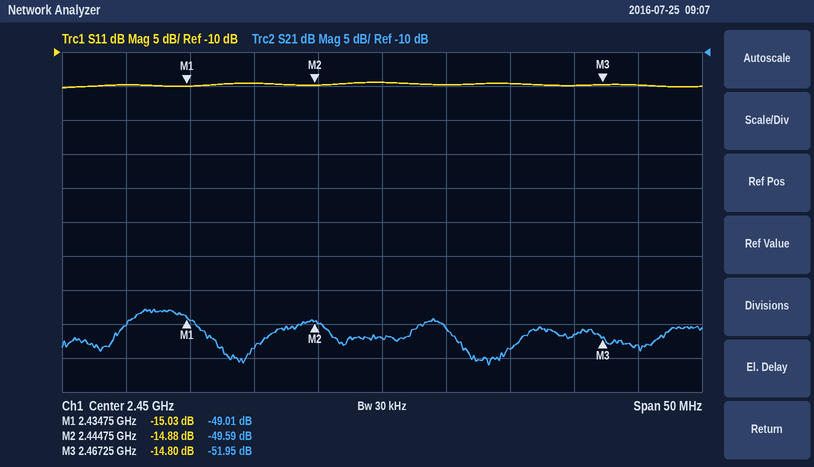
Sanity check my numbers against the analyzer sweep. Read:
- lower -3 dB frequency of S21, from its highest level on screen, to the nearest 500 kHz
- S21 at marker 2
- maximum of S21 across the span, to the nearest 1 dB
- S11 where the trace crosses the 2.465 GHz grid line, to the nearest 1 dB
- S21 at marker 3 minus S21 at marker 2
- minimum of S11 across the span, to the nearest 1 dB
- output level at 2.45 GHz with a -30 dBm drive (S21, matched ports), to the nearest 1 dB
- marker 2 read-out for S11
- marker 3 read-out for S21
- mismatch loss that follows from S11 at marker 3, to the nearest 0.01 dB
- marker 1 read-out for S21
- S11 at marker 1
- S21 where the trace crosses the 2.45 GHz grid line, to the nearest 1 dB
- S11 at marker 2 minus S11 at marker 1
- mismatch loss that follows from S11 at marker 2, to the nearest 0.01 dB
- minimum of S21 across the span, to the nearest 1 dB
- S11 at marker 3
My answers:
2.4295 GHz
-49.59 dB
-48 dB
-15 dB
-2.36 dB
-15 dB
-82 dBm
-14.88 dB
-51.95 dB
0.15 dB
-49.01 dB
-15.03 dB
-52 dB
0.15 dB
0.14 dB
-56 dB
-14.80 dB
